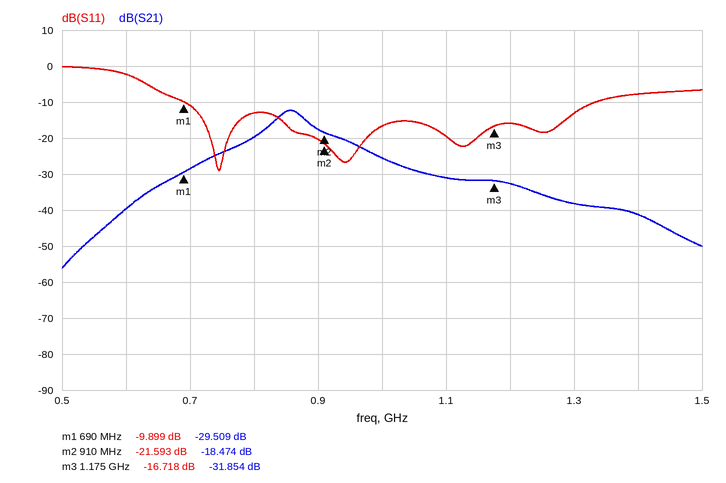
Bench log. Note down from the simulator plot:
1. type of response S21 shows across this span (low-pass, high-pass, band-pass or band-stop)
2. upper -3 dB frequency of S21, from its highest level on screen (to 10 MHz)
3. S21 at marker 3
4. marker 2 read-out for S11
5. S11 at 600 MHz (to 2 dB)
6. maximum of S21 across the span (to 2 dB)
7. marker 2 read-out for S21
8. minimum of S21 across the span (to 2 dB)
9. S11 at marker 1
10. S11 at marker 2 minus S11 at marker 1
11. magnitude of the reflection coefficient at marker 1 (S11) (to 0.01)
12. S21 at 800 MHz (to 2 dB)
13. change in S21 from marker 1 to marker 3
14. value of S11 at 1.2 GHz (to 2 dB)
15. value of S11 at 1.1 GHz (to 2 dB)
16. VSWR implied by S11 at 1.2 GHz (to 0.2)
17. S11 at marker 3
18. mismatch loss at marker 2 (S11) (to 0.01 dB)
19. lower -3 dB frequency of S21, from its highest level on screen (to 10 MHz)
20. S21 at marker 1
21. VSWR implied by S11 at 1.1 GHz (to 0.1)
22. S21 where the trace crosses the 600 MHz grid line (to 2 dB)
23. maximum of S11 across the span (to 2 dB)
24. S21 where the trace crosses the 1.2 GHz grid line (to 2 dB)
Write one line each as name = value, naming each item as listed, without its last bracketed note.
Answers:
type of response S21 shows across this span = band-pass
upper -3 dB frequency of S21, from its highest level on screen = 880 MHz
S21 at marker 3 = -31.854 dB
marker 2 read-out for S11 = -21.593 dB
S11 at 600 MHz = -2 dB
maximum of S21 across the span = -12 dB
marker 2 read-out for S21 = -18.474 dB
minimum of S21 across the span = -56 dB
S11 at marker 1 = -9.899 dB
S11 at marker 2 minus S11 at marker 1 = -11.694 dB
magnitude of the reflection coefficient at marker 1 (S11) = 0.32
S21 at 800 MHz = -20 dB
change in S21 from marker 1 to marker 3 = -2.345 dB
value of S11 at 1.2 GHz = -16 dB
value of S11 at 1.1 GHz = -20 dB
VSWR implied by S11 at 1.2 GHz = 1.4
S11 at marker 3 = -16.718 dB
mismatch loss at marker 2 (S11) = 0.03 dB
lower -3 dB frequency of S21, from its highest level on screen = 830 MHz
S21 at marker 1 = -29.509 dB
VSWR implied by S11 at 1.1 GHz = 1.2
S21 where the trace crosses the 600 MHz grid line = -40 dB
maximum of S11 across the span = 0 dB
S21 where the trace crosses the 1.2 GHz grid line = -32 dB
